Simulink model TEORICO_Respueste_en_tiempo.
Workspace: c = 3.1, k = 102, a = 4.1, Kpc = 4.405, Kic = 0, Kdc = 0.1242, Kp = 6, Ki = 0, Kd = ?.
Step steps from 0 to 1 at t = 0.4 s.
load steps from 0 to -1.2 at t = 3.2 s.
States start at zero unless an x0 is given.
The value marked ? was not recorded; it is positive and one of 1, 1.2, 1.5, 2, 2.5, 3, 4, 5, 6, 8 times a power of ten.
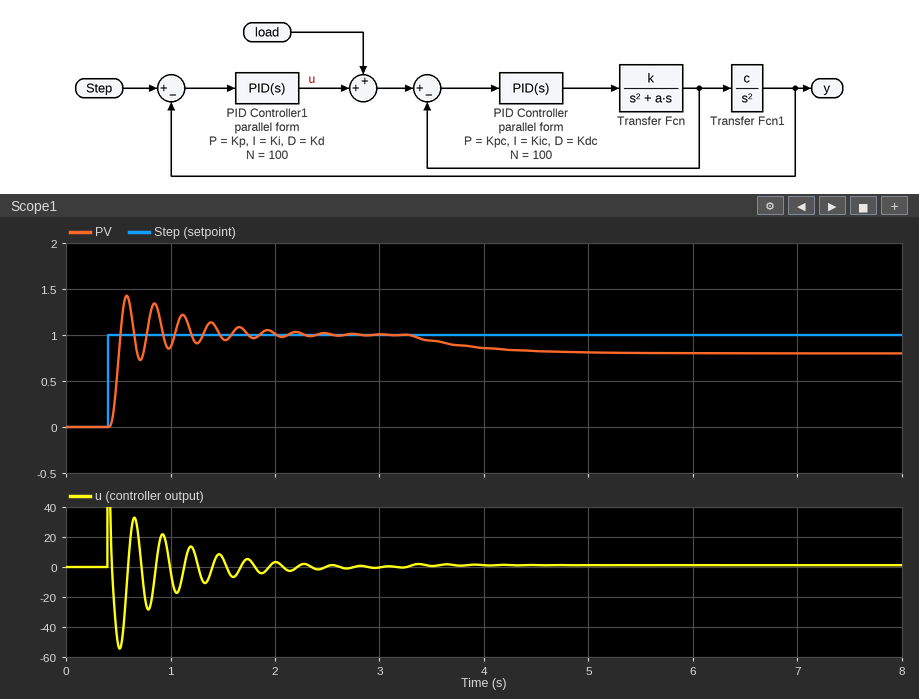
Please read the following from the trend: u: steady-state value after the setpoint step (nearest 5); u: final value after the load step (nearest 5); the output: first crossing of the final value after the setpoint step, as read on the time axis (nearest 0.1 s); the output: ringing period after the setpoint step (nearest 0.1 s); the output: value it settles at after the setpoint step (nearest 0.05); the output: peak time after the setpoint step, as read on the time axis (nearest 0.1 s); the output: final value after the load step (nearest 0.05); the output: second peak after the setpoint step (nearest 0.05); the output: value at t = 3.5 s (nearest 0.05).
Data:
0
0
0.5 s
0.3 s
1.00
0.6 s
0.80
1.35
0.95
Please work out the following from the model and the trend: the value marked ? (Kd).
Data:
4
